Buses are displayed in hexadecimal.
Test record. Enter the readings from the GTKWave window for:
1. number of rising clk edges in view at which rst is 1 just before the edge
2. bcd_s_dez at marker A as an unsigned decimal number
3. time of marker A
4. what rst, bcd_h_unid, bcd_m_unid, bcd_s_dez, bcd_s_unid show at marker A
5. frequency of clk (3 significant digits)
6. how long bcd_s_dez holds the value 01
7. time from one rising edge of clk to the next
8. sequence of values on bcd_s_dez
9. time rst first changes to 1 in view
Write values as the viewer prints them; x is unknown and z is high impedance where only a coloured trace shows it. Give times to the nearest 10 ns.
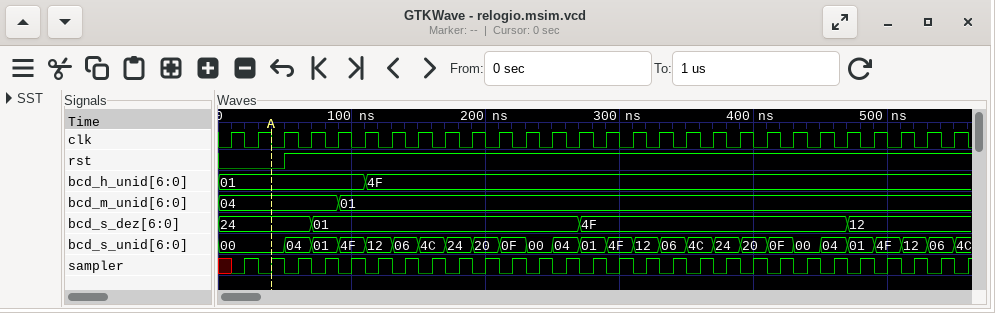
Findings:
25
36
40 ns
rst=0, bcd_h_unid=01, bcd_m_unid=04, bcd_s_dez=24, bcd_s_unid=00
50.0 MHz
200 ns
20 ns
24, 01, 4F, 12
50 ns
